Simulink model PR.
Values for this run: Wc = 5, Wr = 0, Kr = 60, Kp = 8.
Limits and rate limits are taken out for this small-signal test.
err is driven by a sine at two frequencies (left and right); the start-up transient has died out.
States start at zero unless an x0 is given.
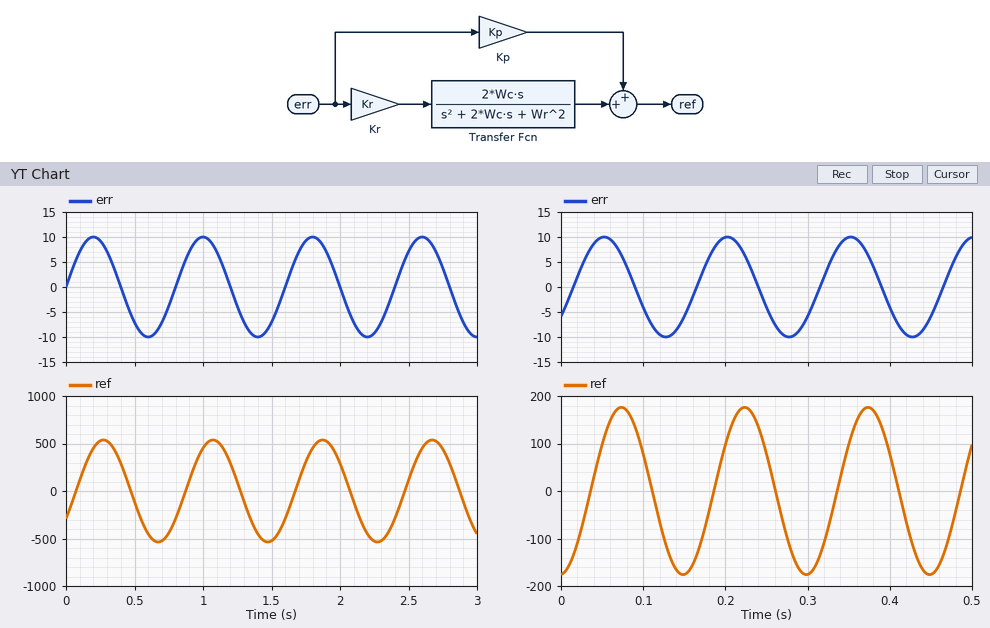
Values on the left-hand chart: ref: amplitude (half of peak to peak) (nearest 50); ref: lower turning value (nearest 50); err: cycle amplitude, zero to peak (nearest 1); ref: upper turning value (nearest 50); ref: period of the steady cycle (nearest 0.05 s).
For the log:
550
-550
10
550
0.80 s
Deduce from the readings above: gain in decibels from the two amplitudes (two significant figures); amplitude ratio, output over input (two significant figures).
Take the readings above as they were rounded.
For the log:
35 dB
55
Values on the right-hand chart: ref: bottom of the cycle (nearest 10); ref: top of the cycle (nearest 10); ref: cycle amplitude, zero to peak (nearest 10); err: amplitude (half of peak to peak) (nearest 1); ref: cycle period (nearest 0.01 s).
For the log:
-180
180
180
10
0.15 s
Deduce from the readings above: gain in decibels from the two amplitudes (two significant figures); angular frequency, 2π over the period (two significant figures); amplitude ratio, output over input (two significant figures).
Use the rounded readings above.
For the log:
25 dB
42 rad/s
18
